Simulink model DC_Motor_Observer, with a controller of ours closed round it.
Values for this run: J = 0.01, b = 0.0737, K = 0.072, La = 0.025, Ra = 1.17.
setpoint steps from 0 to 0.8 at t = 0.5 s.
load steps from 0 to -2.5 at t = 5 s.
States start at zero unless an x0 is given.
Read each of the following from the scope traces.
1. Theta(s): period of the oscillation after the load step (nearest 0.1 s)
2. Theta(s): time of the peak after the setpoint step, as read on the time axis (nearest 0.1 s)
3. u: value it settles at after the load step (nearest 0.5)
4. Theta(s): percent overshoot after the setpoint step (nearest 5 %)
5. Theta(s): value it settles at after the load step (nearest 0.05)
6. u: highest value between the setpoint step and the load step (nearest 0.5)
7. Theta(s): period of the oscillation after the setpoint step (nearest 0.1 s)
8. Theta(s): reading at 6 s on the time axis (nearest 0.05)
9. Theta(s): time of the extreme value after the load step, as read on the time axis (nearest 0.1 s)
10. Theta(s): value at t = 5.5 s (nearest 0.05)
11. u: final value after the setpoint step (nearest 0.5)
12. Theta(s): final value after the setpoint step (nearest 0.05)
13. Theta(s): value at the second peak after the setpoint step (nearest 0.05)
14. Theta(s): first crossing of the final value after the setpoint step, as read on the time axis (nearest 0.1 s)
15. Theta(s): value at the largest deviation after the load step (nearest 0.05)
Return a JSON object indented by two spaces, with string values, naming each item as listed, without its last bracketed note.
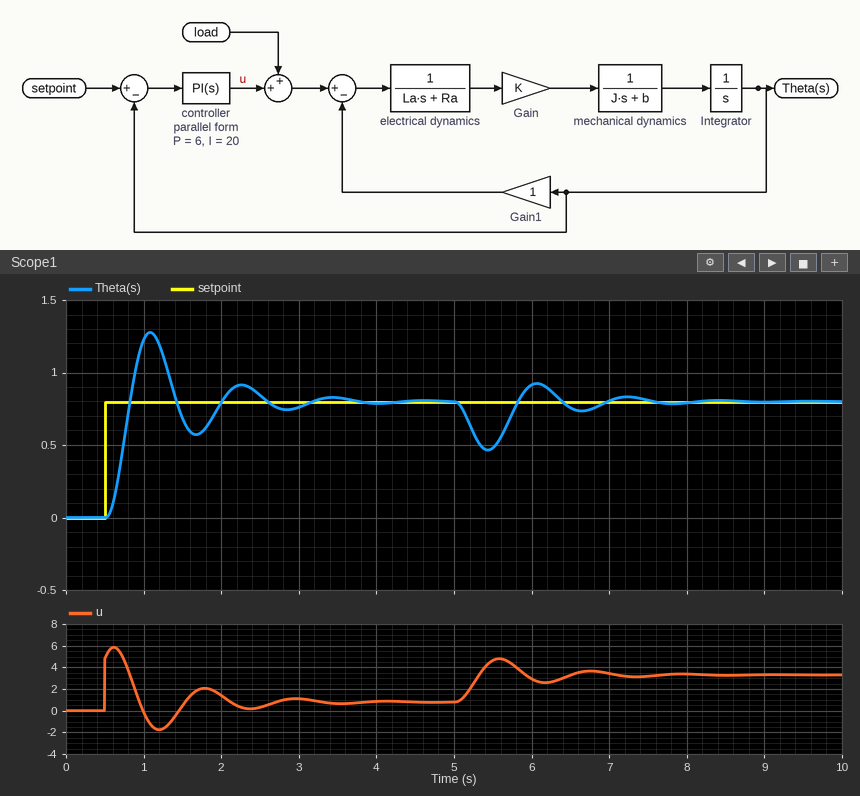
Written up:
{
  "Theta(s): period of the oscillation after the load step": "1.2 s",
  "Theta(s): time of the peak after the setpoint step, as read on the time axis": "1.1 s",
  "u: value it settles at after the load step": "3.5",
  "Theta(s): percent overshoot after the setpoint step": "60 %",
  "Theta(s): value it settles at after the load step": "0.80",
  "u: highest value between the setpoint step and the load step": "6.0",
  "Theta(s): period of the oscillation after the setpoint step": "1.2 s",
  "Theta(s): reading at 6 s on the time axis": "0.90",
  "Theta(s): time of the extreme value after the load step, as read on the time axis": "5.4 s",
  "Theta(s): value at t = 5.5 s": "0.50",
  "u: final value after the setpoint step": "1.0",
  "Theta(s): final value after the setpoint step": "0.80",
  "Theta(s): value at the second peak after the setpoint step": "0.90",
  "Theta(s): first crossing of the final value after the setpoint step, as read on the time axis": "0.8 s",
  "Theta(s): value at the largest deviation after the load step": "0.45"
}
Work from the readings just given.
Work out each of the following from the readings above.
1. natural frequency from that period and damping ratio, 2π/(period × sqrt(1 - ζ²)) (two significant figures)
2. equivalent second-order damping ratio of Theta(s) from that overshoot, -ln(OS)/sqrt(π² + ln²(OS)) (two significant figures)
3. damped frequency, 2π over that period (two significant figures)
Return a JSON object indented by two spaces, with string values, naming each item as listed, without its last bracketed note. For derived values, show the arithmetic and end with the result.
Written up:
{
  "natural frequency from that period and damping ratio, 2π/(period × sqrt(1 - ζ²))": "2π / (1.2 × sqrt(1 - 0.16²)) = 5.3 rad/s",
  "equivalent second-order damping ratio of Theta(s) from that overshoot, -ln(OS)/sqrt(π² + ln²(OS))": "ln(0.6) = -0.511; 0.511 / sqrt(9.870 + 0.261) = 0.16",
  "damped frequency, 2π over that period": "2π / 1.2 = 5.2 rad/s"
}
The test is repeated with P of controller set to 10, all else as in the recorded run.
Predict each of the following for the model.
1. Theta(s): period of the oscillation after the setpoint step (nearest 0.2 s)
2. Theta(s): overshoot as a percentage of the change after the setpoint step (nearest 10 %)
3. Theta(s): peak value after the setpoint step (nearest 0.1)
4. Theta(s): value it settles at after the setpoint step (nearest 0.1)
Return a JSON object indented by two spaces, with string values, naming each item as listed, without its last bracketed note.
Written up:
{
  "Theta(s): period of the oscillation after the setpoint step": "0.8 s",
  "Theta(s): overshoot as a percentage of the change after the setpoint step": "50 %",
  "Theta(s): peak value after the setpoint step": "1.2",
  "Theta(s): value it settles at after the setpoint step": "0.8"
}
